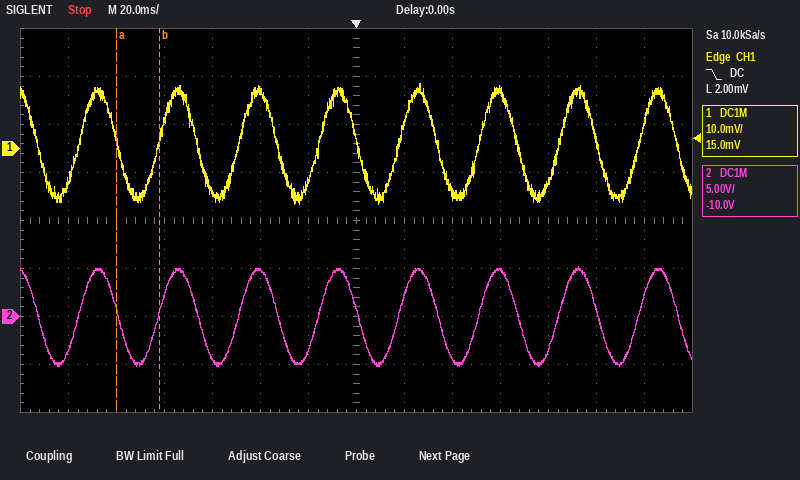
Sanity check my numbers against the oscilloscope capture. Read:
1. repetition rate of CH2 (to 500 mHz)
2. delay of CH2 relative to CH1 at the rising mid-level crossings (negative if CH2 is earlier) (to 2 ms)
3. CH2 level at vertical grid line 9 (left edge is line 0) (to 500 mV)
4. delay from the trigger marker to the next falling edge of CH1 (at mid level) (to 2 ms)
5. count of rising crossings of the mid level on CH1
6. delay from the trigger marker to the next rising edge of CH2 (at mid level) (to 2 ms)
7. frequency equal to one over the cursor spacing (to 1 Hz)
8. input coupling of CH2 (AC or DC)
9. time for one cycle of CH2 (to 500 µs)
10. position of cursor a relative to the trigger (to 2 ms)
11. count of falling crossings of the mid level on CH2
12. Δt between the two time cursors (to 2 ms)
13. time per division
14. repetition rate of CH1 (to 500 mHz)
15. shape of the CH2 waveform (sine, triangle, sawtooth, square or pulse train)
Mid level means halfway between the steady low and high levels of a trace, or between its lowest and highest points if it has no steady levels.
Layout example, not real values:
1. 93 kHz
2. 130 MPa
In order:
1. 30.0 Hz
2. 0 ms
3. -4.5 V
4. 34 ms
5. 8
6. 18 ms
7. 56 Hz
8. DC
9. 33.5 ms
10. -100 ms
11. 9
12. 18 ms
13. 20 ms
14. 30.0 Hz
15. sine
